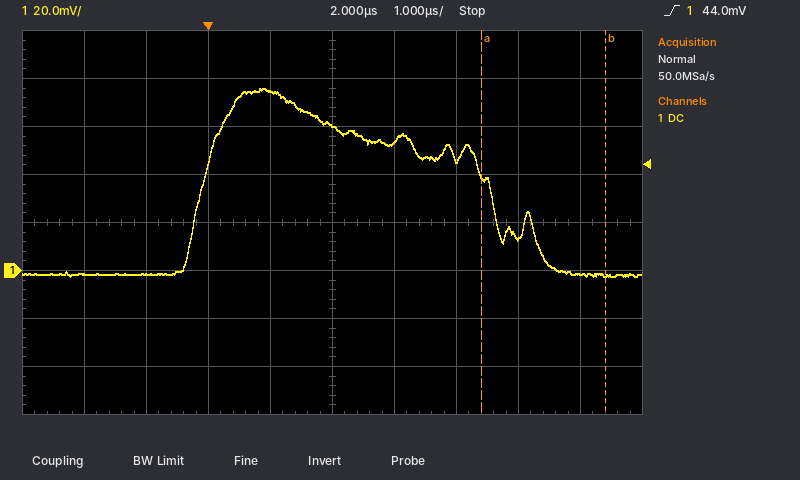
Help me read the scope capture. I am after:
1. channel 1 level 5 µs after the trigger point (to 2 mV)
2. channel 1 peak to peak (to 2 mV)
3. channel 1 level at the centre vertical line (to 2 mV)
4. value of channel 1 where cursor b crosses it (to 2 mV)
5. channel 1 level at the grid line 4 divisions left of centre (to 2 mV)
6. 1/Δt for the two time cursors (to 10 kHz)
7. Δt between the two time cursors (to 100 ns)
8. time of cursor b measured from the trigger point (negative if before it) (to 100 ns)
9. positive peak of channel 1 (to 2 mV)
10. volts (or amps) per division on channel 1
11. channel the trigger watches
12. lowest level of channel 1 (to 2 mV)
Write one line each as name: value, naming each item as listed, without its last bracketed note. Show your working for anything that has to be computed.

channel 1 level 5 µs after the trigger point: 14 mV
channel 1 peak to peak: 76 mV − (-2 mV) = 78 mV
channel 1 level at the centre vertical line: 60 mV
value of channel 1 where cursor b crosses it: -2 mV
channel 1 level at the grid line 4 divisions left of centre: -2 mV
1/Δt for the two time cursors: 1 / 2.0 µs ≈ 500 kHz
Δt between the two time cursors: 2.0 µs
time of cursor b measured from the trigger point (negative if before it): +6.4 µs
positive peak of channel 1: 76 mV
volts (or amps) per division on channel 1: 20 mV
channel the trigger watches: channel 1
lowest level of channel 1: -2 mV
